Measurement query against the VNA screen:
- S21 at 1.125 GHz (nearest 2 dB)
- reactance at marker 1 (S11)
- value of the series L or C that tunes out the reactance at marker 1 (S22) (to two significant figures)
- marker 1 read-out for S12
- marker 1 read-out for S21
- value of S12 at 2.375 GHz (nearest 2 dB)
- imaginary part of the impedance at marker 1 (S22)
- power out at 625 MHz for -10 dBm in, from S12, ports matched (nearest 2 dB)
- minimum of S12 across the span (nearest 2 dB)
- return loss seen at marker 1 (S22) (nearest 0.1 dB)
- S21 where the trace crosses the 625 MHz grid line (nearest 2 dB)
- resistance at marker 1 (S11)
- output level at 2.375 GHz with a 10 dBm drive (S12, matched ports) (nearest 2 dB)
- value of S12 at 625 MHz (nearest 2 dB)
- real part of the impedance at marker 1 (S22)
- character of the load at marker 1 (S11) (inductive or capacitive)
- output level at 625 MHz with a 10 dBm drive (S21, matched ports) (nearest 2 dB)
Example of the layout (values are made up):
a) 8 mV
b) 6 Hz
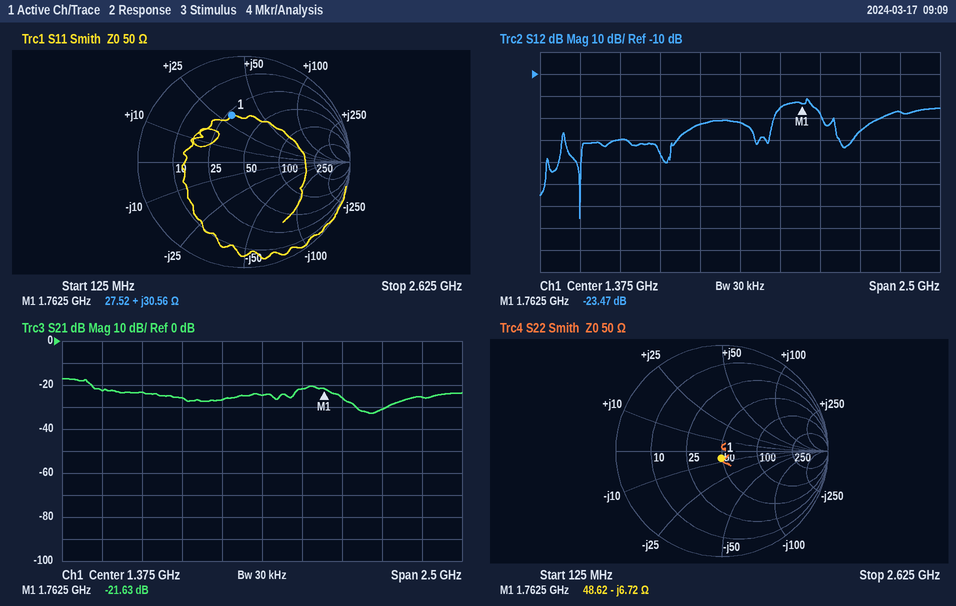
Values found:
a) -26 dB
b) +30.56 Ω
c) 610 pH
d) -23.47 dB
e) -21.63 dB
f) -28 dB
g) -6.72 Ω
h) -50 dBm
i) -76 dB
j) 23.2 dB
k) -24 dB
l) 27.52 Ω
m) -18 dBm
n) -40 dB
o) 48.62 Ω
p) inductive
q) -14 dBm
